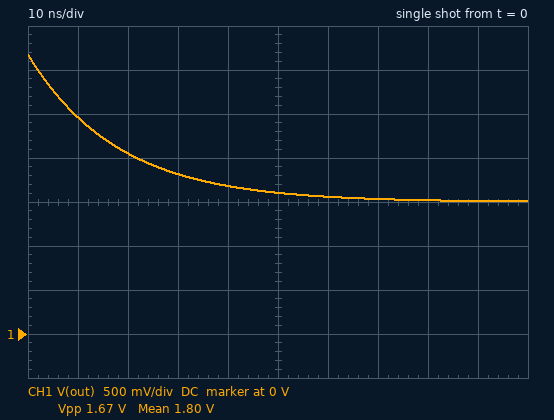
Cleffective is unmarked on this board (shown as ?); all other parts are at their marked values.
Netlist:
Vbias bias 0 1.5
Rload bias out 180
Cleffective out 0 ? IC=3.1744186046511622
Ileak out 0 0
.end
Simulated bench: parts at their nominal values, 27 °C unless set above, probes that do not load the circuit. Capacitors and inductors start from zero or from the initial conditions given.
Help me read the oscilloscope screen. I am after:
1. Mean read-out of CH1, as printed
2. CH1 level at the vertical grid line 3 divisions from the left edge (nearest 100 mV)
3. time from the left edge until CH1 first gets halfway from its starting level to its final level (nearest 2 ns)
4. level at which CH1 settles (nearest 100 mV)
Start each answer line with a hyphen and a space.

- 1.80 V
- 1.8 V
- 12 ns
- 1.5 V
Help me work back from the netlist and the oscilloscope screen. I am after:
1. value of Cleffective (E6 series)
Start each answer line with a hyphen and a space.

- 100 pF
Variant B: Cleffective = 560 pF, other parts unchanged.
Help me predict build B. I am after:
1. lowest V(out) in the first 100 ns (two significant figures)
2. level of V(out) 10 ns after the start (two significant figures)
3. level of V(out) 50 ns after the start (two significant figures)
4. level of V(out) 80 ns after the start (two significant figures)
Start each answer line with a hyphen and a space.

- 2.1 V
- 3.0 V
- 2.5 V
- 2.3 V
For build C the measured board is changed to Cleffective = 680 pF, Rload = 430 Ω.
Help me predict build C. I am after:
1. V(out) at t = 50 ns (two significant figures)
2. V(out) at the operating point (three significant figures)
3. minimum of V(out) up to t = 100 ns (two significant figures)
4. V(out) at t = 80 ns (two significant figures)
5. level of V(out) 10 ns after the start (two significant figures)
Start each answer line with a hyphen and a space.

- 2.9 V
- 1.50 V
- 2.7 V
- 2.8 V
- 3.1 V
